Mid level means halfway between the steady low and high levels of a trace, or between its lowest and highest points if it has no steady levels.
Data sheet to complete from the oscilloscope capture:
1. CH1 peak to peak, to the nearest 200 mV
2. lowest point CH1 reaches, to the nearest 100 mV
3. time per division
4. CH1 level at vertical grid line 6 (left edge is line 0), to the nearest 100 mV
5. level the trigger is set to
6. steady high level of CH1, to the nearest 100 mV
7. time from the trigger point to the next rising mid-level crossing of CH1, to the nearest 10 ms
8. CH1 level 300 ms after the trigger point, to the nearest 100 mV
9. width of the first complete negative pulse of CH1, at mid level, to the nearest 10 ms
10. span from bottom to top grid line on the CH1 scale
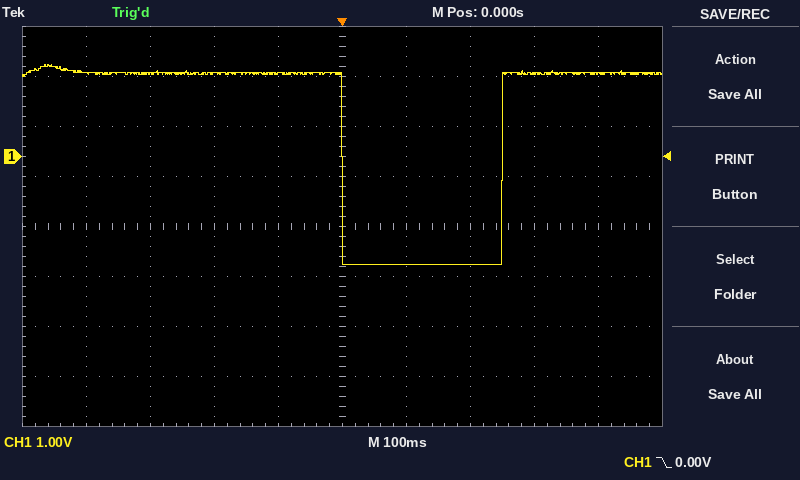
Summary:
4.0 V
-2.2 V
100 ms
-2.2 V
0.00 V
1.7 V
250 ms
1.7 V
250 ms
8 V
